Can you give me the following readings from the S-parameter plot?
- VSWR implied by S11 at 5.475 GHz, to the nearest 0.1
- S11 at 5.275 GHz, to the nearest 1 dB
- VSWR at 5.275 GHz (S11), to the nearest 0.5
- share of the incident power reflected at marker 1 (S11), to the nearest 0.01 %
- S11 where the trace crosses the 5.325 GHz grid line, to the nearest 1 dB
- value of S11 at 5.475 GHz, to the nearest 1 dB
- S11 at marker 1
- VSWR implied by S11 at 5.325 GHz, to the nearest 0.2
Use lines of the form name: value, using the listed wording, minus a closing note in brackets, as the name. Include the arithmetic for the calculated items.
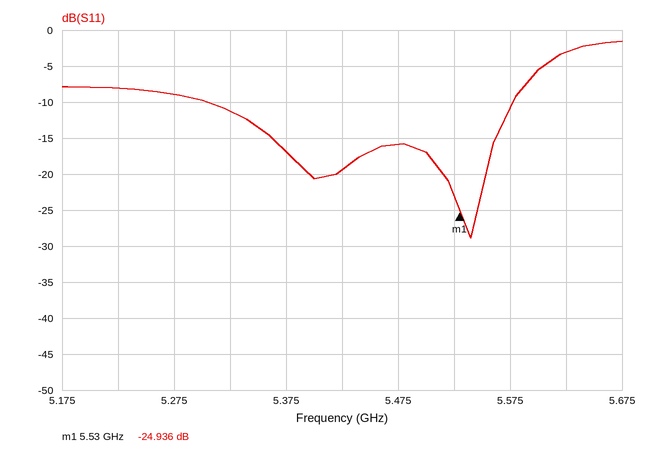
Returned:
VSWR implied by S11 at 5.475 GHz, to the nearest 0.1: |Γ| = 10^(-16/20) = 0.1585; VSWR = (1 + 0.1585)/(1 − 0.1585) ≈ 1.4
S11 at 5.275 GHz, to the nearest 1 dB: -9 dB
VSWR at 5.275 GHz (S11), to the nearest 0.5: |Γ| = 10^(-9/20) = 0.3548; VSWR = (1 + 0.3548)/(1 − 0.3548) ≈ 2.10, so 2.0 to the nearest 0.5
share of the incident power reflected at marker 1 (S11), to the nearest 0.01 %: 10^(-24.936/10) ≈ 0.32 %
S11 where the trace crosses the 5.325 GHz grid line, to the nearest 1 dB: -11 dB
value of S11 at 5.475 GHz, to the nearest 1 dB: -16 dB
S11 at marker 1: -24.936 dB
VSWR implied by S11 at 5.325 GHz, to the nearest 0.2: |Γ| = 10^(-11/20) = 0.2818; VSWR = (1 + 0.2818)/(1 − 0.2818) ≈ 1.8
